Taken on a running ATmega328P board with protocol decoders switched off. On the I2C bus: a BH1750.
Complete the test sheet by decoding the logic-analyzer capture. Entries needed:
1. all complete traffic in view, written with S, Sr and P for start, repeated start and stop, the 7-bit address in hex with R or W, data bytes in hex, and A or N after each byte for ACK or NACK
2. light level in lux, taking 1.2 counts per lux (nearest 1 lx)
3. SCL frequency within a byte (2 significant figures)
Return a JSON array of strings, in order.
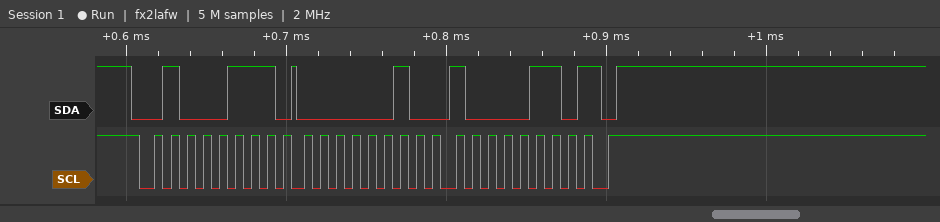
["S 23R A 02 A 86 N P", "538 lx", "100 kHz"]
